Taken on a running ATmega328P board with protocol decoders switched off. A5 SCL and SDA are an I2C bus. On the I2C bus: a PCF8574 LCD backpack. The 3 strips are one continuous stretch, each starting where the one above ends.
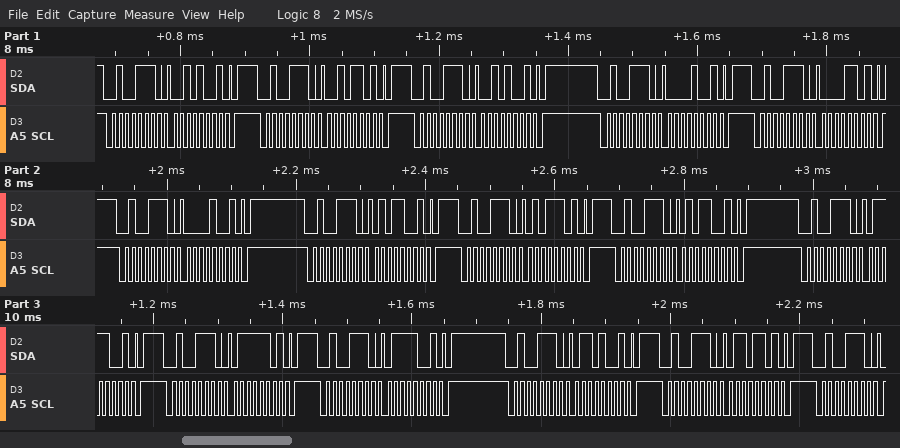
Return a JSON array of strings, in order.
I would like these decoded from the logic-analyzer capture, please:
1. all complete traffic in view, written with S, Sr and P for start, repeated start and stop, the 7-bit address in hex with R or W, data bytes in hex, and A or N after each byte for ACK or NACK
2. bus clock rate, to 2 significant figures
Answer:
["S 27W A 29 A P S 27W A 2D A P S 27W A 29 A P S 27W A 09 A P S 27W A 0D A P S 27W A 09 A P S 27W A 59 A P S 27W A 5D A P S 27W A 59 A P S 27W A 79 A P S 27W A 7D A P S 27W A 79 A P S 27W A 69 A P S 27W A 6D A P S 27W A", "100 kHz"]
